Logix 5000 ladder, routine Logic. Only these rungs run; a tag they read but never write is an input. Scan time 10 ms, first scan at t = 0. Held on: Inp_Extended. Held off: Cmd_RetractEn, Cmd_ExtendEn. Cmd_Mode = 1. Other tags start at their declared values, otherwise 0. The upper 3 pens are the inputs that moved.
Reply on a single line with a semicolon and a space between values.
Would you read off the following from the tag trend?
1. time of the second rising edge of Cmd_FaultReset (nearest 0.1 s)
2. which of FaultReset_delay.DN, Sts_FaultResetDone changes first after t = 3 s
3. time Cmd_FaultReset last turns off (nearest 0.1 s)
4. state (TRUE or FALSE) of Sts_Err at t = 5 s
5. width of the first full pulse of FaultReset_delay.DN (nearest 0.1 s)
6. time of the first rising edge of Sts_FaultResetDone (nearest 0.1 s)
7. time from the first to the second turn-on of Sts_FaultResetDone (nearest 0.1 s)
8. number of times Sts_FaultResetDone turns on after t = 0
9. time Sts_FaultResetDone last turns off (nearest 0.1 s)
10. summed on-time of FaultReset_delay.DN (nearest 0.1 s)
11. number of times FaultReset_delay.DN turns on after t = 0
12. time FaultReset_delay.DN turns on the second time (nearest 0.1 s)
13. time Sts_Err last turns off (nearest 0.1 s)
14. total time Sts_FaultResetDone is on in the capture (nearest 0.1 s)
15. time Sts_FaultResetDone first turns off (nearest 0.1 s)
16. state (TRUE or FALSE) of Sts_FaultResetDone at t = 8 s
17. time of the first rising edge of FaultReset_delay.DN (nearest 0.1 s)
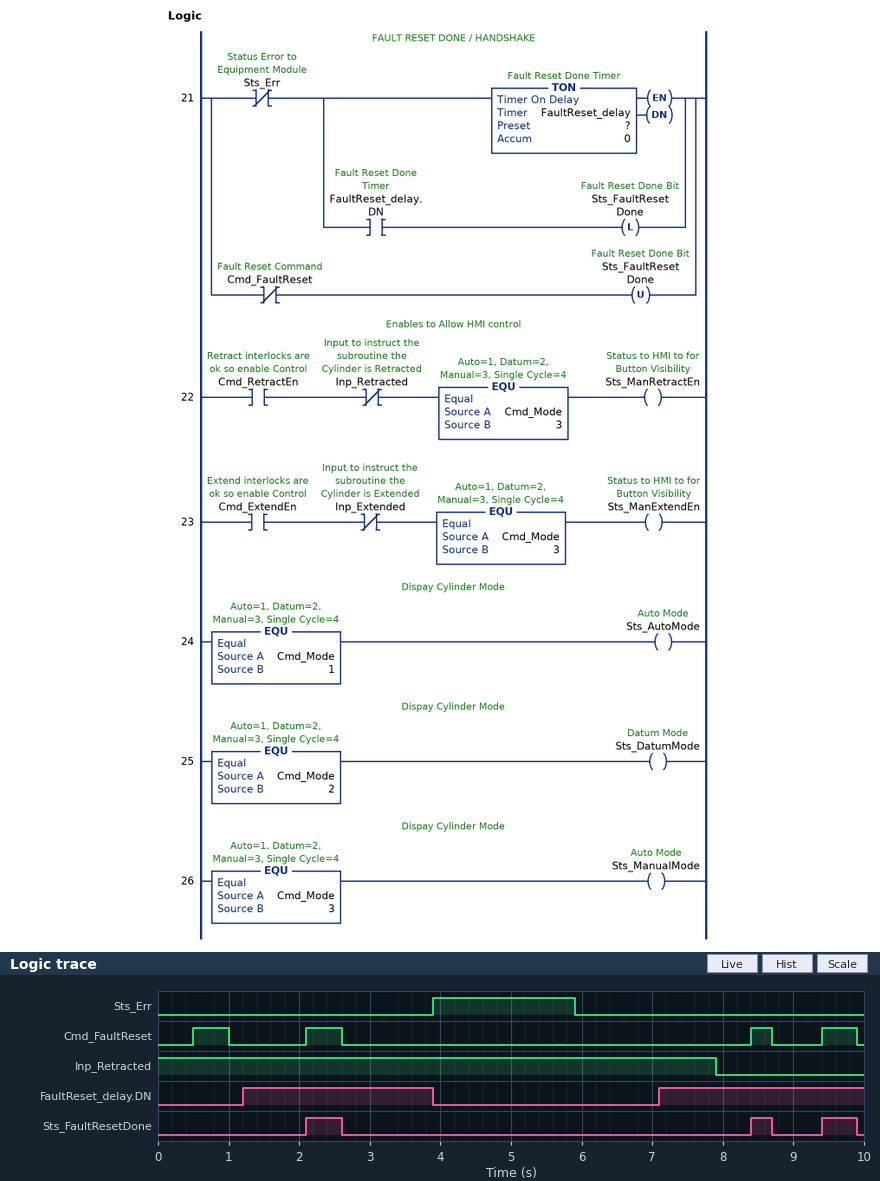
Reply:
2.1 s; FaultReset_delay.DN; 9.9 s; TRUE; 2.7 s; 2.1 s; 6.3 s; 3; 9.9 s; 5.6 s; 2; 7.1 s; 5.9 s; 1.3 s; 2.6 s; FALSE; 1.2 s
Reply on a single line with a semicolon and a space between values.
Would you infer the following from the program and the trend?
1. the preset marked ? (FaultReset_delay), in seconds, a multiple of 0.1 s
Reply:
1.2 s
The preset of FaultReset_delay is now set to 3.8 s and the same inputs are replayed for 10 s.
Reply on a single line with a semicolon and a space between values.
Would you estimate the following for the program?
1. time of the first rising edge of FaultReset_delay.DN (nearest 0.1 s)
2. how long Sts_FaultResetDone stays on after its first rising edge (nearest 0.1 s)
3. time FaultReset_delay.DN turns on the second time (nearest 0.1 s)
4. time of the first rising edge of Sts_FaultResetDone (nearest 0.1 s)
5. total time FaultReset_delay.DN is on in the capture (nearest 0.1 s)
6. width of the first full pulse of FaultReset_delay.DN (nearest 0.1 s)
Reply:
3.8 s; 0.2 s; 9.7 s; 9.7 s; 0.4 s; 0.1 s
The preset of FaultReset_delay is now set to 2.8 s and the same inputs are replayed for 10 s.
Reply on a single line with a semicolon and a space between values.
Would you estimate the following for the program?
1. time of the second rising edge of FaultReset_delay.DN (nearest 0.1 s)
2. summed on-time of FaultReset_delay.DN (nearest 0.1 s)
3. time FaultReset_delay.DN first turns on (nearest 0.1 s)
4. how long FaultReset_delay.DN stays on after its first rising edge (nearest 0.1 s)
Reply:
8.7 s; 2.4 s; 2.8 s; 1.1 s
